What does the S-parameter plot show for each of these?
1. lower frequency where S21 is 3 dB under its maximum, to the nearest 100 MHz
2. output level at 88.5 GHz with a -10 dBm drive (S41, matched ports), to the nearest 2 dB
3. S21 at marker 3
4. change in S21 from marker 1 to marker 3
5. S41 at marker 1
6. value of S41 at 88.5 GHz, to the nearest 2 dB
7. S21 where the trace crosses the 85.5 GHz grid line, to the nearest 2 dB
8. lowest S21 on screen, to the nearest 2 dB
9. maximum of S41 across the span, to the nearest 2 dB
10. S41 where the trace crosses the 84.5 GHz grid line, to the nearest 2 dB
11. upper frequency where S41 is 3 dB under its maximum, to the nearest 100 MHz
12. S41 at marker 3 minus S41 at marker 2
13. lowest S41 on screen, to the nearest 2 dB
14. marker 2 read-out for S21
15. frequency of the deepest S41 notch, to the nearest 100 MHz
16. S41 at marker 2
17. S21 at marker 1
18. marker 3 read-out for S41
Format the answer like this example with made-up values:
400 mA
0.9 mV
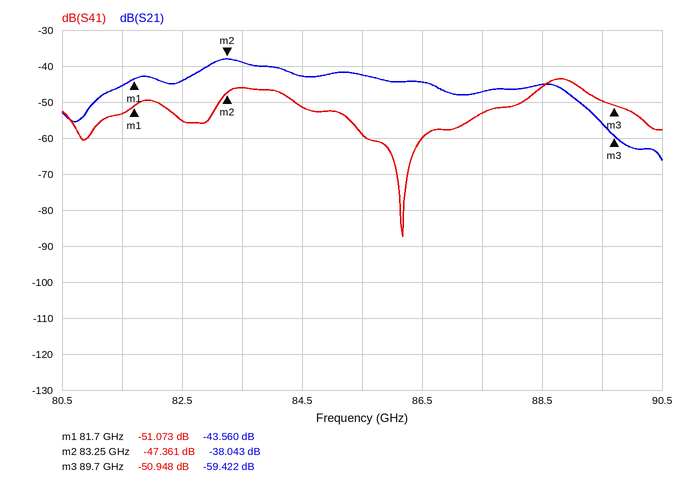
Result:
82.8 GHz
-56 dBm
-59.422 dB
-15.862 dB
-51.073 dB
-46 dB
-42 dB
-66 dB
-44 dB
-52 dB
89.2 GHz
-3.587 dB
-88 dB
-38.043 dB
86.2 GHz
-47.361 dB
-43.560 dB
-50.948 dB
